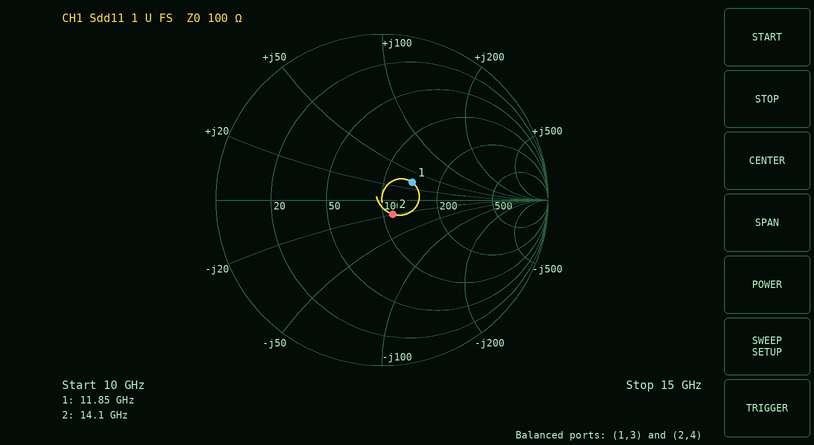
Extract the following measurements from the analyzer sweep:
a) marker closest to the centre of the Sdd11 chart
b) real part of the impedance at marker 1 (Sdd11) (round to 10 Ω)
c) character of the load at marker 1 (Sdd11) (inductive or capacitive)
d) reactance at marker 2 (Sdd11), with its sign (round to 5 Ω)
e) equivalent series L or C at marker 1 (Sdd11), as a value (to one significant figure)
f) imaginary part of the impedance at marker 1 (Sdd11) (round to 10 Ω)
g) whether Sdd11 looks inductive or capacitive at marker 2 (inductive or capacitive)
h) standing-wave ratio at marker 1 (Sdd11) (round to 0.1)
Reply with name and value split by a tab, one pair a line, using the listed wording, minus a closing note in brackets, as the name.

marker closest to the centre of the Sdd11 chart	marker 2
real part of the impedance at marker 1 (Sdd11)	140 Ω
character of the load at marker 1 (Sdd11)	inductive
reactance at marker 2 (Sdd11), with its sign	-20 Ω
equivalent series L or C at marker 1 (Sdd11), as a value	400 pH
imaginary part of the impedance at marker 1 (Sdd11)	+30 Ω
whether Sdd11 looks inductive or capacitive at marker 2	capacitive
standing-wave ratio at marker 1 (Sdd11)	1.5
